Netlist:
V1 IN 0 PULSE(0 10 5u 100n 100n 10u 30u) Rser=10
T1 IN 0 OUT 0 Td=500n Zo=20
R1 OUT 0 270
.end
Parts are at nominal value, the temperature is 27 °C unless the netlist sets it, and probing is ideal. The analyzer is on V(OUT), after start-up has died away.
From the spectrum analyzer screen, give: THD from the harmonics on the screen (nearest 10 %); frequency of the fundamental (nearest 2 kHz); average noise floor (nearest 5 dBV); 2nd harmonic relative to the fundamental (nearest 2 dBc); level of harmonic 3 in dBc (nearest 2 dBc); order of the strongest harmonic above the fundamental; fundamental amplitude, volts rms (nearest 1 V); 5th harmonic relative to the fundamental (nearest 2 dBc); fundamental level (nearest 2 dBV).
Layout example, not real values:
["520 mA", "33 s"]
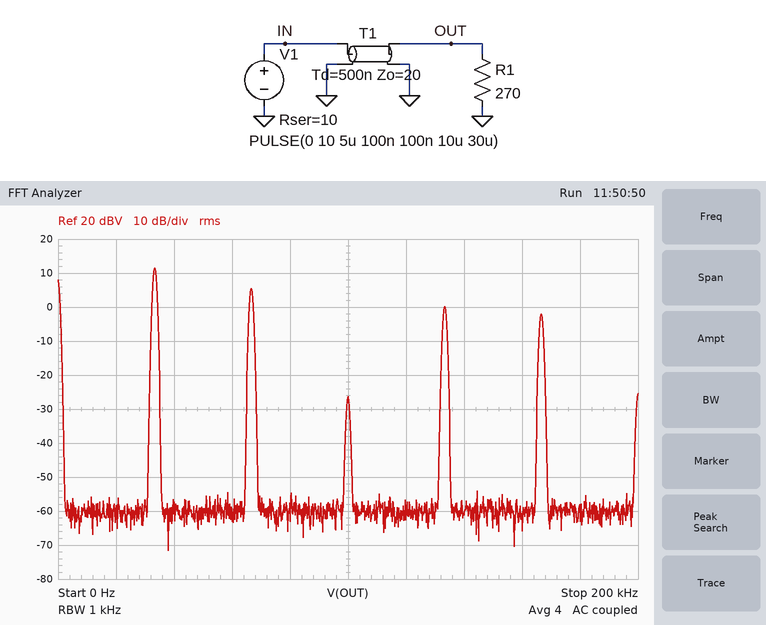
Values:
["60 %", "34 kHz", "-60 dBV", "-6 dBc", "-38 dBc", "2", "4 V", "-14 dBc", "12 dBV"]
